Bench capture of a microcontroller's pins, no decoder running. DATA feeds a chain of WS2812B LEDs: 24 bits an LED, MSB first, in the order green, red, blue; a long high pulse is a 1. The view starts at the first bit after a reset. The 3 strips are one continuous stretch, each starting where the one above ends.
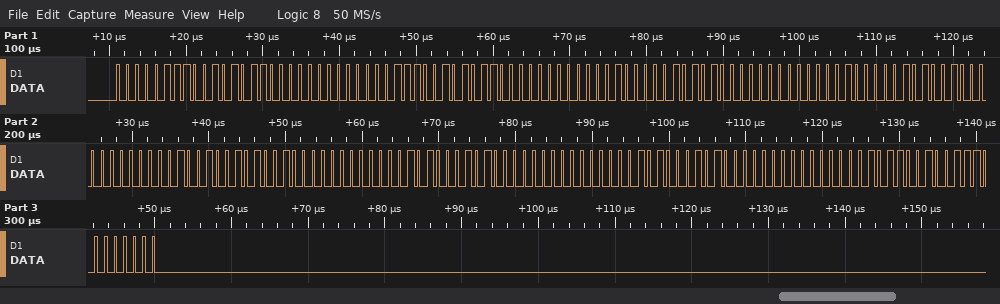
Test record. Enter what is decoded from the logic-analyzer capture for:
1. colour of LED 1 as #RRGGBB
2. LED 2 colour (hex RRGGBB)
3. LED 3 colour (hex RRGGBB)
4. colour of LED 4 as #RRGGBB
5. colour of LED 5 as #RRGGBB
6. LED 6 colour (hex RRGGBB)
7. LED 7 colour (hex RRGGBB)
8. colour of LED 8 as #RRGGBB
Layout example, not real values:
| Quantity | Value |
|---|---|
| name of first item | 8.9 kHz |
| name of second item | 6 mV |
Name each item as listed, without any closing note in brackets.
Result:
| Quantity | Value |
|---|---|
| colour of LED 1 as #RRGGBB | #2B0700 |
| LED 2 colour | #2B0700 |
| LED 3 colour | #2A0800 |
| colour of LED 4 as #RRGGBB | #290800 |
| colour of LED 5 as #RRGGBB | #290900 |
| LED 6 colour | #280A00 |
| LED 7 colour | #280A00 |
| colour of LED 8 as #RRGGBB | #270B00 |
